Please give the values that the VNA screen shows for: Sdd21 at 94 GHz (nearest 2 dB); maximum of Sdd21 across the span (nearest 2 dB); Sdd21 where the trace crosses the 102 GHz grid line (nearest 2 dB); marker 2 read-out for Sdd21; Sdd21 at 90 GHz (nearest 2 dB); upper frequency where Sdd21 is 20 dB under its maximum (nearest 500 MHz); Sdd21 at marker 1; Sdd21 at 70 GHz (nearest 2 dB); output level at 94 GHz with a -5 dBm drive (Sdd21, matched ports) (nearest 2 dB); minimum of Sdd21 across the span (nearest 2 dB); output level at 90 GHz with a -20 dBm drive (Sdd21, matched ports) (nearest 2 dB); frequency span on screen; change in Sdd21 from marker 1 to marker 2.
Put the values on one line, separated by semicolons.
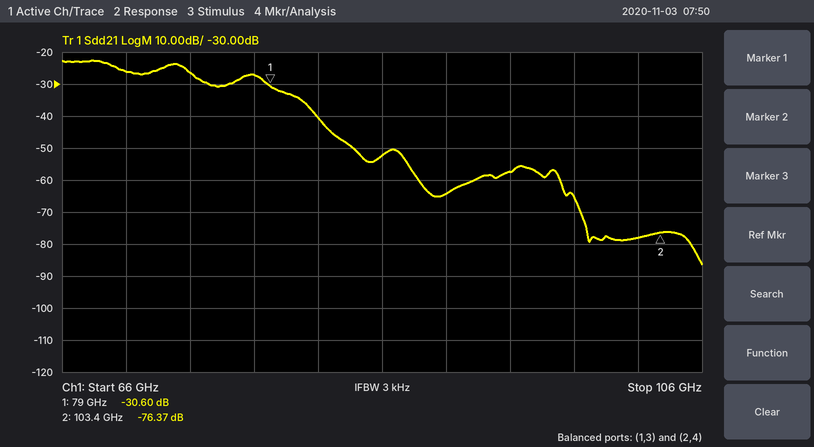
-58 dB; -22 dB; -78 dB; -76.37 dB; -64 dB; 82.5 GHz; -30.60 dB; -26 dB; -62 dBm; -86 dB; -84 dBm; 40 GHz; -45.77 dB
